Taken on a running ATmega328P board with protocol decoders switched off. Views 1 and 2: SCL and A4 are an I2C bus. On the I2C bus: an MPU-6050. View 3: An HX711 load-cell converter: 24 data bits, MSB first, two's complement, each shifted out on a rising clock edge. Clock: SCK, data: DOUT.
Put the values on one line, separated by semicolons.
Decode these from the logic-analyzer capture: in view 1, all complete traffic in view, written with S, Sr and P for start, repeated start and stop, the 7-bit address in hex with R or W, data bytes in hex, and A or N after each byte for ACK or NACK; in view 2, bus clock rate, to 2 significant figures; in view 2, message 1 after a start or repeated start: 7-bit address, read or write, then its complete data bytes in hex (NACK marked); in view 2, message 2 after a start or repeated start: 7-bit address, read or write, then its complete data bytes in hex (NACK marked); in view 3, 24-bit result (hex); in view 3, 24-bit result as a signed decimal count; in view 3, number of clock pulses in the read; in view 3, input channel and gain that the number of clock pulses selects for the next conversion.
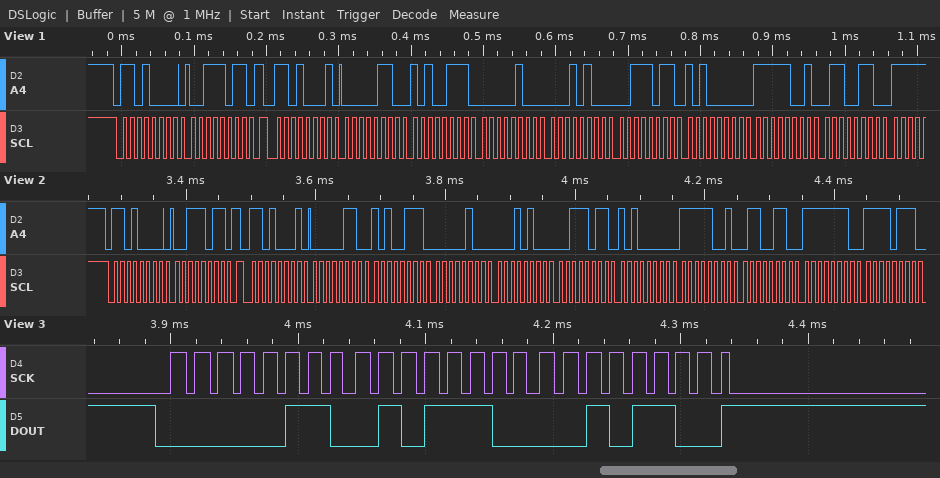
S 68W A 3B A Sr 68R A 06 A A7 A 04 A 14 A 3B A A0 A F9 A 66 A; 100 kHz; 0x68 write: 3B; 0x68 read: 06 A7 04 14 3B A0 F9 66 FE F7; 0x065C2C; 416812; 25; channel A, gain 128
